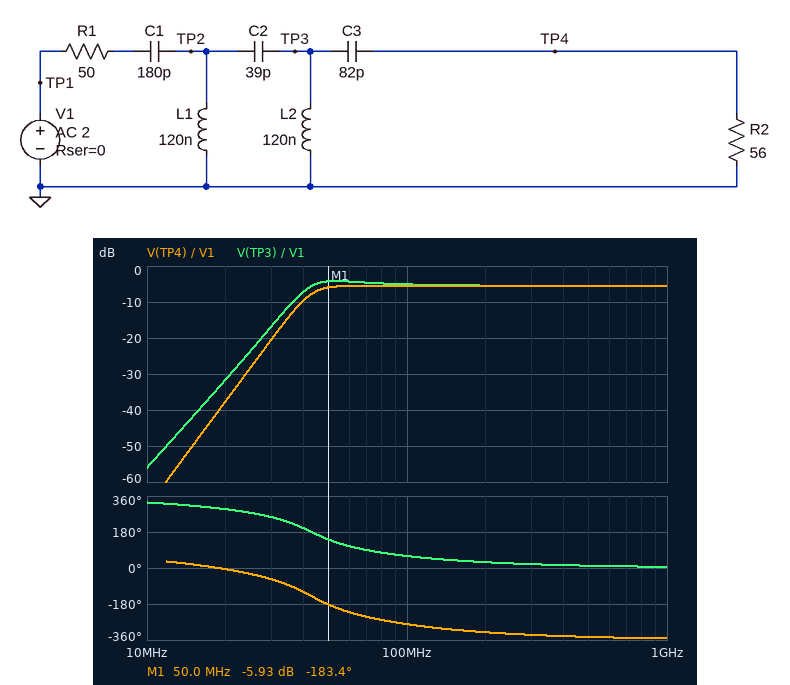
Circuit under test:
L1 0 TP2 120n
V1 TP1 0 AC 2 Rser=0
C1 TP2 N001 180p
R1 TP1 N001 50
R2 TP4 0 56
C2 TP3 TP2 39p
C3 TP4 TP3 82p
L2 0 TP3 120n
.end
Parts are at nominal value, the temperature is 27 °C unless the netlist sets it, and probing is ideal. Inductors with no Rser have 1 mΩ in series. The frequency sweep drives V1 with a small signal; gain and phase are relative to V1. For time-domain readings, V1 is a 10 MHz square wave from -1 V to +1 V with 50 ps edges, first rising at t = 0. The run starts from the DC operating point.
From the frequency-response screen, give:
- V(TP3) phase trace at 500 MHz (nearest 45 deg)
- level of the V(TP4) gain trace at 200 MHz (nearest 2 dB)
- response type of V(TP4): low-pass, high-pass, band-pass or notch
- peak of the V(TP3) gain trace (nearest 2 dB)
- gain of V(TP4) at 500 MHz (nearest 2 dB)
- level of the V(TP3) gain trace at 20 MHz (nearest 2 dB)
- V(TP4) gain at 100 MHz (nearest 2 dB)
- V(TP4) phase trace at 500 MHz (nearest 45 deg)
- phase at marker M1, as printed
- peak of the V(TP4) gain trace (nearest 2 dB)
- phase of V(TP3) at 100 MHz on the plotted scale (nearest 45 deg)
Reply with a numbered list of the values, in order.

1. 0 deg
2. -6 dB
3. high-pass
4. -4 dB
5. -6 dB
6. -32 dB
7. -6 dB
8. -360 deg
9. -183.4 deg
10. -6 dB
11. 45 deg
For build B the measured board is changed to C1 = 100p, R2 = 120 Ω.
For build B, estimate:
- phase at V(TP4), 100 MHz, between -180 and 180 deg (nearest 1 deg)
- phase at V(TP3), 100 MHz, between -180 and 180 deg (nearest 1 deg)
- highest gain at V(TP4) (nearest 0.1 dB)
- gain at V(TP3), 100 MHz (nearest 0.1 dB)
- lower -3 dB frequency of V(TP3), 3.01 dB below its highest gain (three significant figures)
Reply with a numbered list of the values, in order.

1. 82 deg
2. 73 deg
3. -2.9 dB
4. -2.8 dB
5. 42.3 MHz
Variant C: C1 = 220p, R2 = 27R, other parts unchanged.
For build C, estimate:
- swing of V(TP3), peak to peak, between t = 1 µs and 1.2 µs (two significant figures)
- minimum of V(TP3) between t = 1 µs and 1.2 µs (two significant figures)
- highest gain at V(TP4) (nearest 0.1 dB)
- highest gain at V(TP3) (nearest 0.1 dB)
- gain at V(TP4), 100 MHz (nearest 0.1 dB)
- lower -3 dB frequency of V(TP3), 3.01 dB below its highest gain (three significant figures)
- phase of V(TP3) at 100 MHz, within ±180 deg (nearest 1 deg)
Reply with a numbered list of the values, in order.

1. 1.4 V
2. -700 mV
3. -9.0 dB
4. -3.9 dB
5. -9.2 dB
6. 36.7 MHz
7. 45 deg
